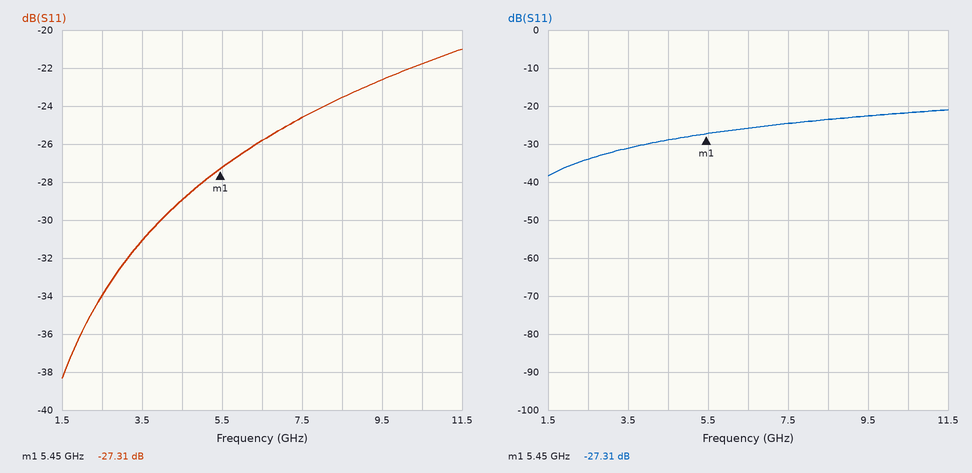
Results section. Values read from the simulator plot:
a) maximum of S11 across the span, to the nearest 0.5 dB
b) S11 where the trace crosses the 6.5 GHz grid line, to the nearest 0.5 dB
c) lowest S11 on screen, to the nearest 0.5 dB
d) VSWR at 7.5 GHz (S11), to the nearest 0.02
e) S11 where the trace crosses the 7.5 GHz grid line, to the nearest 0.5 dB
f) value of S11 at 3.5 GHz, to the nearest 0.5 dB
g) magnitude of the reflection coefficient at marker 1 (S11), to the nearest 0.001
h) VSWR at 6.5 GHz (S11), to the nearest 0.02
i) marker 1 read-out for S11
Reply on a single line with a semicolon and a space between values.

-21.0 dB; -26.0 dB; -38.5 dB; 1.12; -24.5 dB; -31.0 dB; 0.043; 1.10; -27.31 dB
